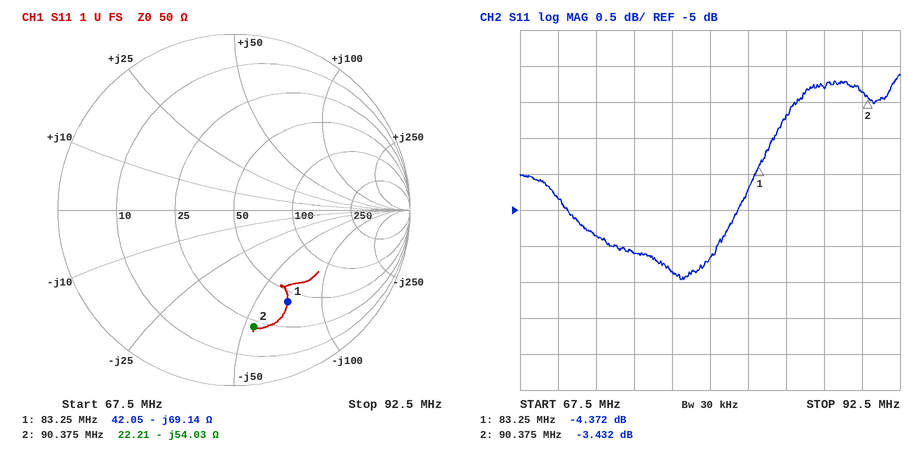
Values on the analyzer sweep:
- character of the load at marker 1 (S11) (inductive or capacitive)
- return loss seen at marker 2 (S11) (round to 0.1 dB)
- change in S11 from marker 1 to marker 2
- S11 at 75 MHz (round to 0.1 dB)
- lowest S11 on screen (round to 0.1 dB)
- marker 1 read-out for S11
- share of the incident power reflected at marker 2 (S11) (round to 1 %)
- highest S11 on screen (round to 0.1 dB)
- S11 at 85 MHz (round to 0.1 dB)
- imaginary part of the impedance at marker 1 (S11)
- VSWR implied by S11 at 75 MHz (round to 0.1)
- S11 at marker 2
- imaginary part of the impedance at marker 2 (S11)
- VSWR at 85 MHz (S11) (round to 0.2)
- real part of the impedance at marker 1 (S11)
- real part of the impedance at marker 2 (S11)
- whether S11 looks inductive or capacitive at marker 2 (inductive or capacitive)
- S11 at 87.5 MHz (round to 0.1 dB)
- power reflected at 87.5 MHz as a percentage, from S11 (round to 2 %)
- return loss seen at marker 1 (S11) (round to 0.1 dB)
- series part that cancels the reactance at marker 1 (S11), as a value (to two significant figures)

capacitive
3.4 dB
0.940 dB
-5.6 dB
-6.0 dB
-4.372 dB
45 %
-3.1 dB
-3.7 dB
-69.14 Ω
3.2
-3.432 dB
-54.03 Ω
4.8
42.05 Ω
22.21 Ω
capacitive
-3.3 dB
46 %
4.4 dB
130 nH
